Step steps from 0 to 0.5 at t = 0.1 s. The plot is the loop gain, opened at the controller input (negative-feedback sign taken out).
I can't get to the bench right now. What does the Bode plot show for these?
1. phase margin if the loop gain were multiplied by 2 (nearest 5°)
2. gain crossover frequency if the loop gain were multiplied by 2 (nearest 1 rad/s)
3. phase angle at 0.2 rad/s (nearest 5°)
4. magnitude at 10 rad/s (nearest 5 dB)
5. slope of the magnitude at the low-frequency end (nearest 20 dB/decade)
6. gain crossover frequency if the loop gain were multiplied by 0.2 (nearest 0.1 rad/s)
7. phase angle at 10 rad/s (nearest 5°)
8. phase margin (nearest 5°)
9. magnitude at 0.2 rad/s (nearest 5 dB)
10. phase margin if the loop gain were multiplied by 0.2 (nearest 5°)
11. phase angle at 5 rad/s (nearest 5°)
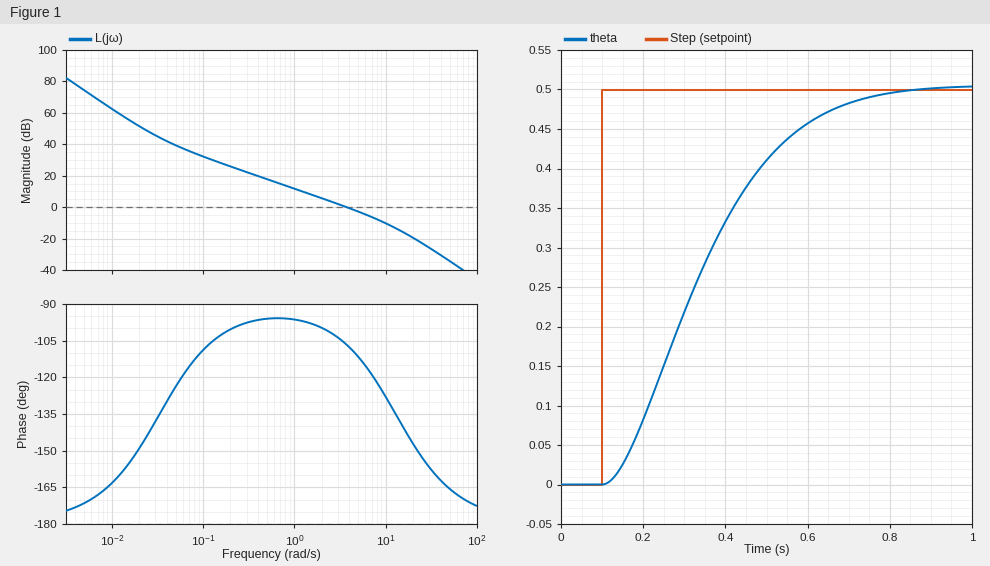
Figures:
60°
7 rad/s
-100°
-10 dB
-40 dB/decade
0.8 rad/s
-130°
75°
25 dB
85°
-110°
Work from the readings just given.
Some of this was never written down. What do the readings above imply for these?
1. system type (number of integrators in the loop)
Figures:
2
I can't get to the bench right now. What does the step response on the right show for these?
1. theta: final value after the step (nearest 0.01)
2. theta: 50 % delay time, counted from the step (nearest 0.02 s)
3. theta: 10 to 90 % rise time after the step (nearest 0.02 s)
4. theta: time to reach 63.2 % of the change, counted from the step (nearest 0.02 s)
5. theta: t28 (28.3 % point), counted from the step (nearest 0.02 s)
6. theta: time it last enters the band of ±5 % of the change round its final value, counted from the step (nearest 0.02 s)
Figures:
0.50
0.22 s
0.42 s
0.28 s
0.14 s
0.58 s
